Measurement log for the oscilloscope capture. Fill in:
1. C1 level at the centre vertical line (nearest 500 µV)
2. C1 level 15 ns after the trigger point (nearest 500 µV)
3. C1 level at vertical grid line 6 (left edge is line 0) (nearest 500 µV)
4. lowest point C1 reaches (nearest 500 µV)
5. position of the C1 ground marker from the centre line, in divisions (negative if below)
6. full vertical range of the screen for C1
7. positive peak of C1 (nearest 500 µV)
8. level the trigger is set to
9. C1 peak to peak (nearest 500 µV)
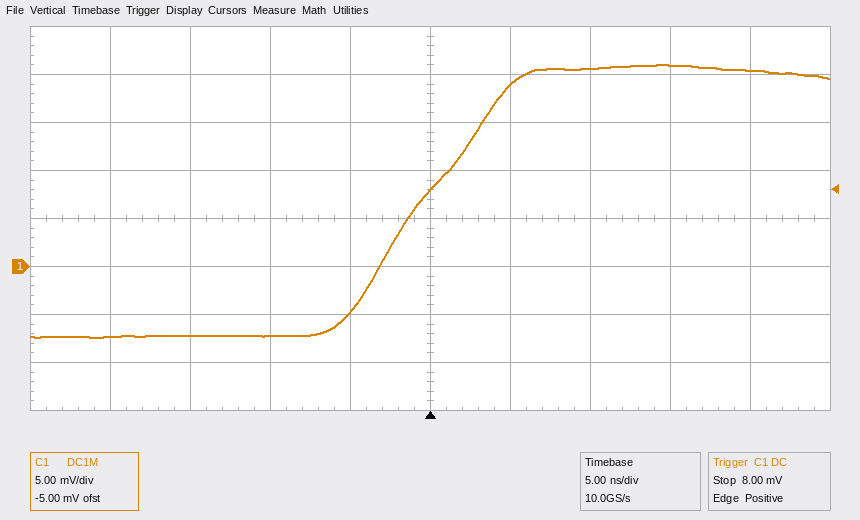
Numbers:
8.0 mV
21.0 mV
19.0 mV
-7.5 mV
-1.0 div
40 mV
21.0 mV
8.00 mV
28.5 mV
